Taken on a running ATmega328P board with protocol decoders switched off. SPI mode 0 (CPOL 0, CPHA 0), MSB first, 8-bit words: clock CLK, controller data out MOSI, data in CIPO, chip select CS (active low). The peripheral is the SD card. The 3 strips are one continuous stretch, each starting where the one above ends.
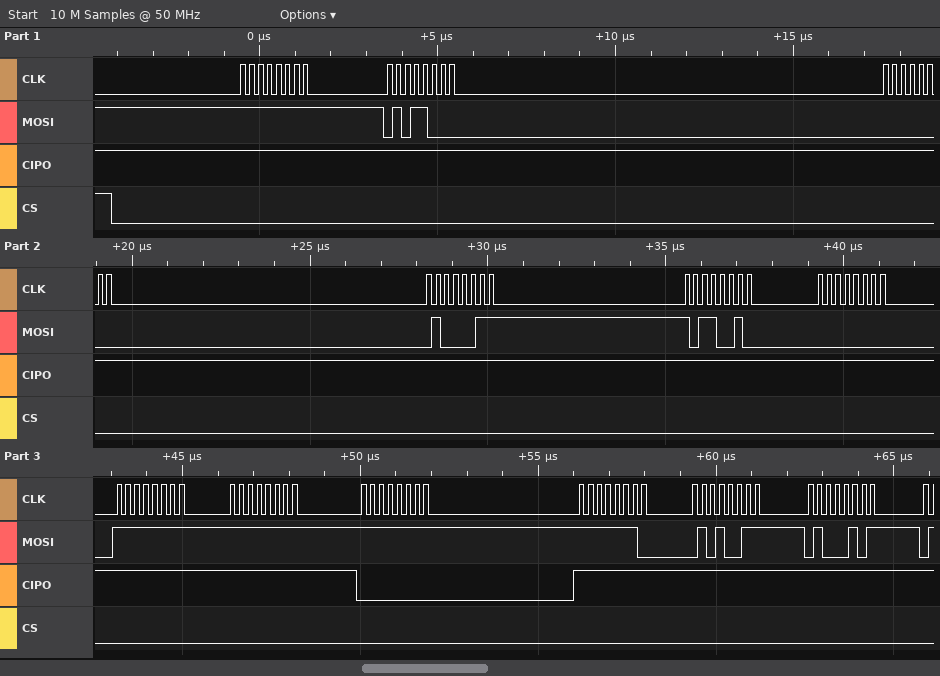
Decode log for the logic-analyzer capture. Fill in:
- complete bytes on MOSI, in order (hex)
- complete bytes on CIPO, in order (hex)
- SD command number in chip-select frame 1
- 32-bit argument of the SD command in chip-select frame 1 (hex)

0xFF 0x58 0x00 0x43 0xB2 0x00 0xFF 0xFF 0xFF 0xFE 0x53 0x45
0xFF 0xFF 0xFF 0xFF 0xFF 0xFF 0xFF 0xFF 0x00 0xFF 0xFF 0xFF
CMD24
0x0043B200
